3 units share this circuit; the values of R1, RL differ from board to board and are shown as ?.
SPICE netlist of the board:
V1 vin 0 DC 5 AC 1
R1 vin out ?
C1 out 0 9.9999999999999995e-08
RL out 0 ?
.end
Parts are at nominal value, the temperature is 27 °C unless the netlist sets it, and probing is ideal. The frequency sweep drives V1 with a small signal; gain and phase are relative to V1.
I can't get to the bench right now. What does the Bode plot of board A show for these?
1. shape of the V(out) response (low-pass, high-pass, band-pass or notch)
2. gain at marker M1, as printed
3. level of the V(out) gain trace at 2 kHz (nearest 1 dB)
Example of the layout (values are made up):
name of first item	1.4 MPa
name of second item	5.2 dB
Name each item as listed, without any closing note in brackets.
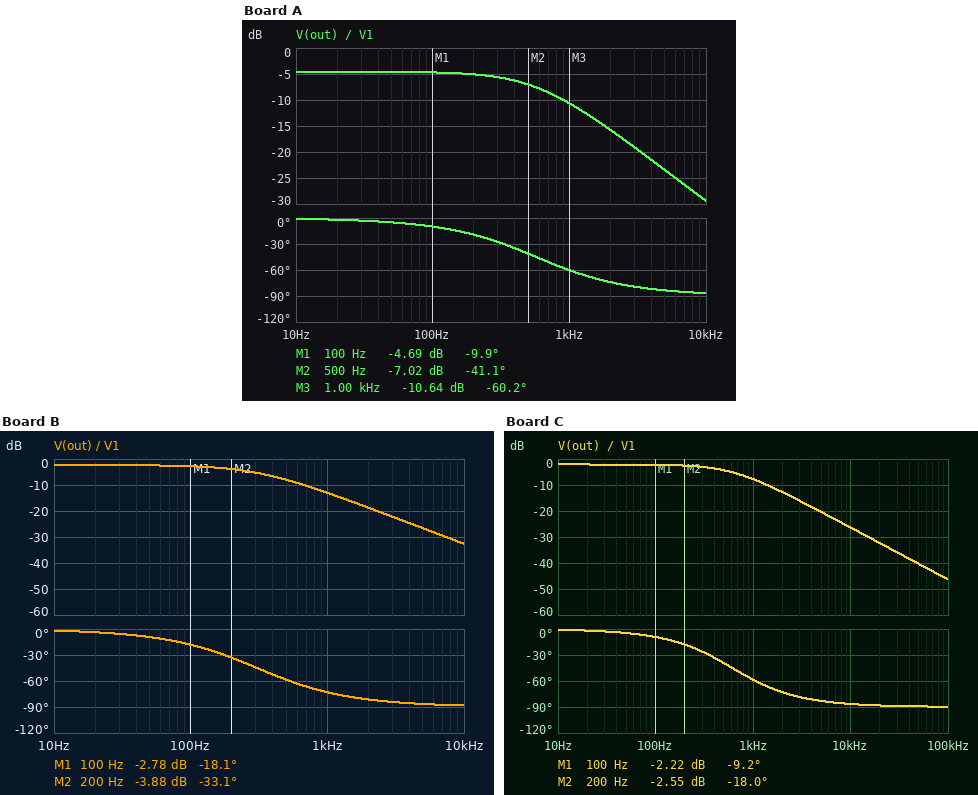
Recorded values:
shape of the V(out) response	low-pass
gain at marker M1, as printed	-4.69 dB
level of the V(out) gain trace at 2 kHz	-16 dB
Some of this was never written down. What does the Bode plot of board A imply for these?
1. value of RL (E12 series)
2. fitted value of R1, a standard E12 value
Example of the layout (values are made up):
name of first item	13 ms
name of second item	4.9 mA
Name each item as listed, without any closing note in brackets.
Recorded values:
value of RL	6.8 kΩ
fitted value of R1, a standard E12 value	4.7 kΩ
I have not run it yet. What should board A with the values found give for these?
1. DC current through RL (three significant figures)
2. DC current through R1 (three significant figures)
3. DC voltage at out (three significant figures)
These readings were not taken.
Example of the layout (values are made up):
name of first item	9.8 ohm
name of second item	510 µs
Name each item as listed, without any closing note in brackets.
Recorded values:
DC current through RL	435 µA
DC current through R1	435 µA
DC voltage at out	2.96 V
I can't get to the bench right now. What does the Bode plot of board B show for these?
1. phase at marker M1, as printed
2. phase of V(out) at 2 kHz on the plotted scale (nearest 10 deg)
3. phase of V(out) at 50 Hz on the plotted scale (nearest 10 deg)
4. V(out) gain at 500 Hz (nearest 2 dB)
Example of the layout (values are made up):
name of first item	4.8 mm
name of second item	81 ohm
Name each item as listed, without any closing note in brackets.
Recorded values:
phase at marker M1, as printed	-18.1 deg
phase of V(out) at 2 kHz on the plotted scale	-80 deg
phase of V(out) at 50 Hz on the plotted scale	-10 deg
V(out) gain at 500 Hz	-8 dB
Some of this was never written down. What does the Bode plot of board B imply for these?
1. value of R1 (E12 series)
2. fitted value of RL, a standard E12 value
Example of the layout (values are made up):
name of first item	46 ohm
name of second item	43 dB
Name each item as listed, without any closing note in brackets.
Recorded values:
value of R1	6.8 kΩ
fitted value of RL, a standard E12 value	22 kΩ
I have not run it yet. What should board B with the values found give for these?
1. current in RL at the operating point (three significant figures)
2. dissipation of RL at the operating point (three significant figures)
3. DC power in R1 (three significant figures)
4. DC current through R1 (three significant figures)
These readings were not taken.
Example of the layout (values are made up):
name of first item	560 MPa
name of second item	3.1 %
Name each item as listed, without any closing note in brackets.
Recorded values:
current in RL at the operating point	174 µA
dissipation of RL at the operating point	663 µW
DC power in R1	205 µW
DC current through R1	174 µA
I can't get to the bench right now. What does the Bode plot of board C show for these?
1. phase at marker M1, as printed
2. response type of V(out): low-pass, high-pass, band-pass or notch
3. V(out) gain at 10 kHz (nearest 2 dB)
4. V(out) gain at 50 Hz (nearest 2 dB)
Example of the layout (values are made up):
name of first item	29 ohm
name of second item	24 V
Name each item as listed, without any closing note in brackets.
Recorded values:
phase at marker M1, as printed	-9.2 deg
response type of V(out): low-pass, high-pass, band-pass or notch	low-pass
V(out) gain at 10 kHz	-26 dB
V(out) gain at 50 Hz	-2 dB
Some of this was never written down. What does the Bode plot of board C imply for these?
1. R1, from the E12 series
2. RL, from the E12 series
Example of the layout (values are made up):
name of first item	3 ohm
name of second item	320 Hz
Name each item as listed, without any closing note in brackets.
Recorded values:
R1, from the E12 series	3.3 kΩ
RL, from the E12 series	12 kΩ
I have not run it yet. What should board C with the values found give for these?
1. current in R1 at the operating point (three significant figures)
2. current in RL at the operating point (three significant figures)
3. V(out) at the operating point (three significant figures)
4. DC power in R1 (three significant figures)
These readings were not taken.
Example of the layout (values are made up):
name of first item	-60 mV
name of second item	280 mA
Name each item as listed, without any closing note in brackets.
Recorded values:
current in R1 at the operating point	327 µA
current in RL at the operating point	327 µA
V(out) at the operating point	3.92 V
DC power in R1	352 µW
